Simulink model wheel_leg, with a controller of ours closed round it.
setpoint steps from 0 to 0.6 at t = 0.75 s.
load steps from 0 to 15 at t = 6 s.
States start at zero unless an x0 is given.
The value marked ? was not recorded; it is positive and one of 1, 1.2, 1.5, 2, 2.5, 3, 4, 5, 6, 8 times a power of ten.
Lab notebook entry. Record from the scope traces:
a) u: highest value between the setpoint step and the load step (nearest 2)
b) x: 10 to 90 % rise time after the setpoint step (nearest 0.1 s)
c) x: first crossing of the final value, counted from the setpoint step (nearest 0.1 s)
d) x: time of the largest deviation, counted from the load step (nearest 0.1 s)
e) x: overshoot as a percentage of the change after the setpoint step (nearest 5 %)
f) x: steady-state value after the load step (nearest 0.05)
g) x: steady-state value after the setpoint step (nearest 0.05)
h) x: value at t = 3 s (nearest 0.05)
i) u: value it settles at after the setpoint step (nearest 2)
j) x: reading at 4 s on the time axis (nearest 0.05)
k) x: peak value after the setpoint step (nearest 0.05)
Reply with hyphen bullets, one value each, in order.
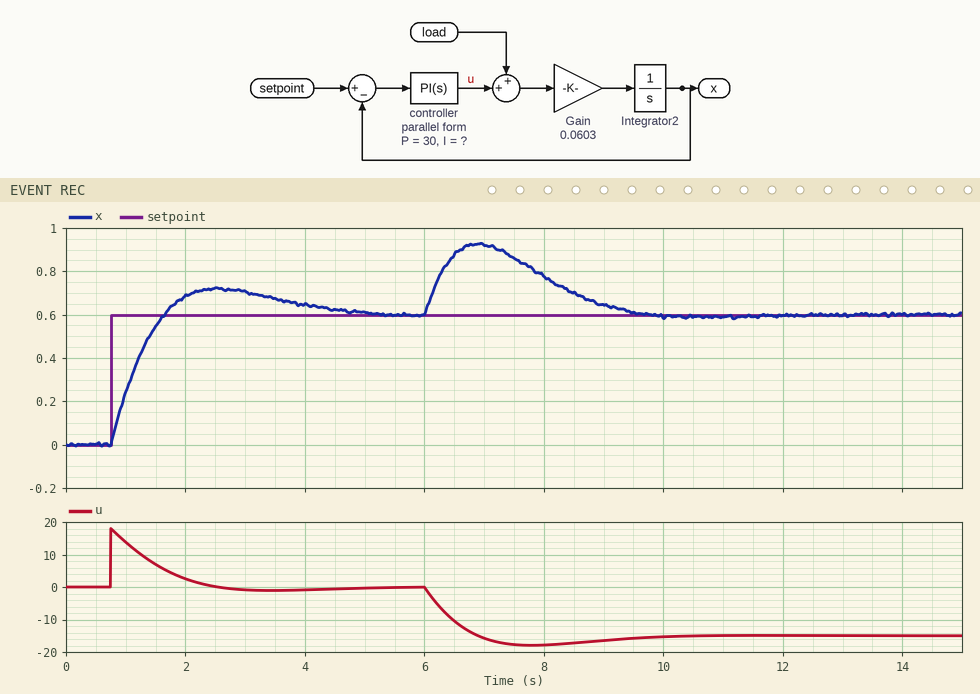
- 18
- 0.7 s
- 0.9 s
- 0.9 s
- 20 %
- 0.60
- 0.60
- 0.70
- 0
- 0.65
- 0.70
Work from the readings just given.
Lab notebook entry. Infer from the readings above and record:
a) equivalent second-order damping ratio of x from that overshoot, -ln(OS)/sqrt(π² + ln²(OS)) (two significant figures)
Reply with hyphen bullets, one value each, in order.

- 0.46
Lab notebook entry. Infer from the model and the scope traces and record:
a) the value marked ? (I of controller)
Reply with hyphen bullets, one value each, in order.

- 25
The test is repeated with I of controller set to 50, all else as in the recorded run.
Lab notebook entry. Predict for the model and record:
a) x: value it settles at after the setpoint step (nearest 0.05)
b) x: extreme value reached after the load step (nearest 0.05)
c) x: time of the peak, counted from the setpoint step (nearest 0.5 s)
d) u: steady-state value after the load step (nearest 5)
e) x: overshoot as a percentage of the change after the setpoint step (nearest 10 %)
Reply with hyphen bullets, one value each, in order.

- 0.60
- 0.90
- 1.5 s
- -15
- 30 %
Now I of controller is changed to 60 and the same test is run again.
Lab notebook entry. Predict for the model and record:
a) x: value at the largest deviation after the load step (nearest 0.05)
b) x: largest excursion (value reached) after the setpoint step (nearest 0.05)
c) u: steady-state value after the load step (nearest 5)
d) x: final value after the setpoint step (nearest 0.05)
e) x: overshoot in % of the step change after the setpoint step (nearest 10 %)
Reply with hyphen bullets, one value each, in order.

- 0.85
- 0.80
- -15
- 0.60
- 30 %
